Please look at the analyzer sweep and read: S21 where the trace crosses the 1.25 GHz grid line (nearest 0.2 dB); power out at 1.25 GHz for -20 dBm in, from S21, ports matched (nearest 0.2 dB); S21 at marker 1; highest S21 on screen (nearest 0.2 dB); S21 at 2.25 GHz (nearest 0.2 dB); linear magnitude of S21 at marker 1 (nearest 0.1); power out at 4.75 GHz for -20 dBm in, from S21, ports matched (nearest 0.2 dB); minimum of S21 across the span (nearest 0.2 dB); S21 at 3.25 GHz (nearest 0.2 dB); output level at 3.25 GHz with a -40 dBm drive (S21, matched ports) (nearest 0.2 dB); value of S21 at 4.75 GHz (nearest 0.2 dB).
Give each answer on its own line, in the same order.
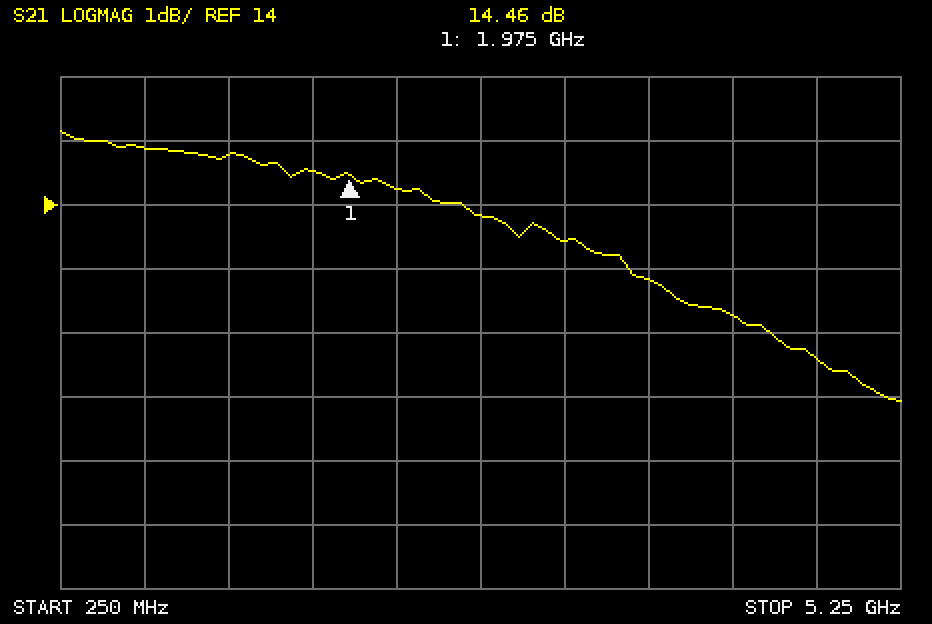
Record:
14.8 dB
-5.2 dBm
14.46 dB
15.2 dB
14.2 dB
5.3
-8.4 dBm
11.0 dB
13.4 dB
-26.6 dBm
11.6 dB
